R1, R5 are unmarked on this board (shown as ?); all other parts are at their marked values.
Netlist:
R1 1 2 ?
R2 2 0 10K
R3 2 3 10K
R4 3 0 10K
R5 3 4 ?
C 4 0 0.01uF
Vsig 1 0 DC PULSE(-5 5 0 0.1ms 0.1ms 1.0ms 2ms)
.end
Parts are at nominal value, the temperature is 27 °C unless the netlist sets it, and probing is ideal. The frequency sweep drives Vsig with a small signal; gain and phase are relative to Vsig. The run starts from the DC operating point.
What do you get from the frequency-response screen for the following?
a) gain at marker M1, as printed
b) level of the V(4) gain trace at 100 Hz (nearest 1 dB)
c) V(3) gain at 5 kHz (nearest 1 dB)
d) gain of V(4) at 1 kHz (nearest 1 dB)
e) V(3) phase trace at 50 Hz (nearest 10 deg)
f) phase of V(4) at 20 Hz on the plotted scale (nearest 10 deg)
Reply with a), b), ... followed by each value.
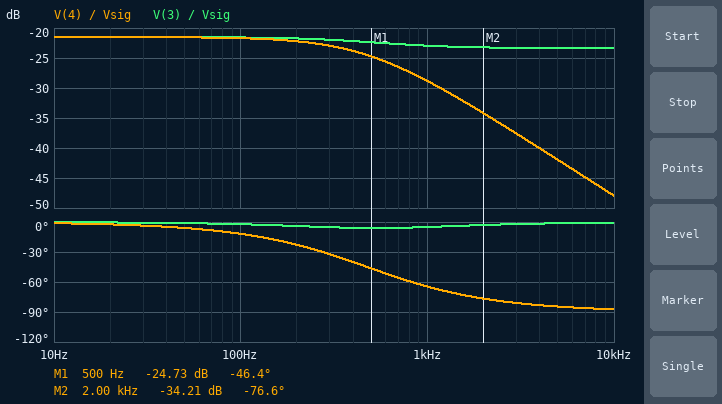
a) -24.73 dB
b) -22 dB
c) -23 dB
d) -29 dB
e) 0 deg
f) 0 deg
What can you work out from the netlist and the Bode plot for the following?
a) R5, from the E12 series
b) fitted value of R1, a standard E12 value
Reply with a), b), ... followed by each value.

a) 27 kΩ
b) 33 kΩ
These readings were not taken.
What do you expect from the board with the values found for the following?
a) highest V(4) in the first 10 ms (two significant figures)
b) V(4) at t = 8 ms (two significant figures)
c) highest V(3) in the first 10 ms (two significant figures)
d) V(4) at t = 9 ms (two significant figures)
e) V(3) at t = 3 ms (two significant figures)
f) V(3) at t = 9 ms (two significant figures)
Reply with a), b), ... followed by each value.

a) 390 mV
b) -360 mV
c) 410 mV
d) 370 mV
e) 410 mV
f) 410 mV
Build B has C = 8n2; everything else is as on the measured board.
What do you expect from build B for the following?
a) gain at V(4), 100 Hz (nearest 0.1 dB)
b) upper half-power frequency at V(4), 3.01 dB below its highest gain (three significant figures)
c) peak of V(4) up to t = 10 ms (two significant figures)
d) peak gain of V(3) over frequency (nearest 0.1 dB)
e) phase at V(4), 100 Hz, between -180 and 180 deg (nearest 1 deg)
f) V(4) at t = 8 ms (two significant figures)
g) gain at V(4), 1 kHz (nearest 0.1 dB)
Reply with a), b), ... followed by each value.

a) -21.6 dB
b) 581 Hz
c) 400 mV
d) -21.5 dB
e) -10 deg
f) -380 mV
g) -27.5 dB
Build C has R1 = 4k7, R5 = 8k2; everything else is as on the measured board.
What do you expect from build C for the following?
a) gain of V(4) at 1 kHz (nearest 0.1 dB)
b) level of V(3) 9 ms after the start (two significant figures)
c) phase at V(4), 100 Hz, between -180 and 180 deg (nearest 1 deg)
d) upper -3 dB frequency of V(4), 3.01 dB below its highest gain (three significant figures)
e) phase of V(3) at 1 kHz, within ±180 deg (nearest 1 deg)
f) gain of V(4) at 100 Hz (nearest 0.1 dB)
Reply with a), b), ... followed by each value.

a) -13.1 dB
b) 1.5 V
c) -5 deg
d) 1.15 kHz
e) -14 deg
f) -10.7 dB
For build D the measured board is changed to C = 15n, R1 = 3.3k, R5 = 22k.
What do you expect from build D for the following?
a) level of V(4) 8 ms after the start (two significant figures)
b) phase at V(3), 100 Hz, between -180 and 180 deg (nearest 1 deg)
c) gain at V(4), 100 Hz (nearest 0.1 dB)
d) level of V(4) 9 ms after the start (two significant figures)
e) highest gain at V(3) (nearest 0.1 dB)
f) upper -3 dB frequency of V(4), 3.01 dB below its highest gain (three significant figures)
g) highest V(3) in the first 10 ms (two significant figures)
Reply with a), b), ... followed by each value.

a) -1.3 V
b) -3 deg
c) -9.8 dB
d) 1.4 V
e) -9.5 dB
f) 385 Hz
g) 1.6 V
